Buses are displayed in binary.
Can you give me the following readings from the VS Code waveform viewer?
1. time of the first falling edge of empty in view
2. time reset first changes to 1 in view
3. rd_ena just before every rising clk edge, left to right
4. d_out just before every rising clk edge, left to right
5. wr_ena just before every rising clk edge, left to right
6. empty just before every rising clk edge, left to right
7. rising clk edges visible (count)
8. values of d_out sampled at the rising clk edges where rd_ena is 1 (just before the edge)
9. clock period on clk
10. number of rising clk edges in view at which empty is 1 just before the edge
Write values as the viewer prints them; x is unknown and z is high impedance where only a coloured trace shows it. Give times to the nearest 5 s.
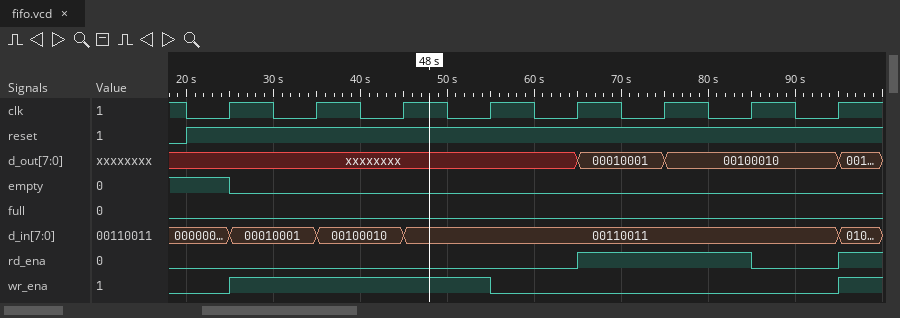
25 s
20 s
0 0 0 0 0 1 1 0
xxxxxxxx, xxxxxxxx, xxxxxxxx, xxxxxxxx, xxxxxxxx, 00010001, 00100010, 00100010
0 1 1 1 0 0 0 0
1 0 0 0 0 0 0 0
8
00010001, 00100010
10 s
1
